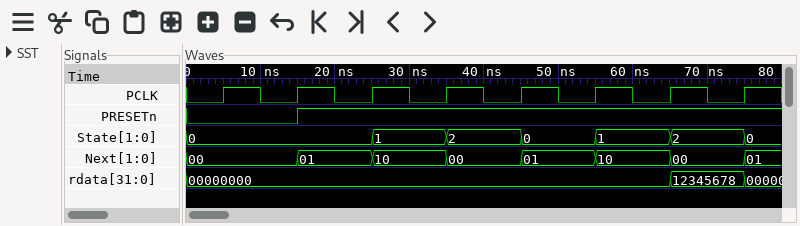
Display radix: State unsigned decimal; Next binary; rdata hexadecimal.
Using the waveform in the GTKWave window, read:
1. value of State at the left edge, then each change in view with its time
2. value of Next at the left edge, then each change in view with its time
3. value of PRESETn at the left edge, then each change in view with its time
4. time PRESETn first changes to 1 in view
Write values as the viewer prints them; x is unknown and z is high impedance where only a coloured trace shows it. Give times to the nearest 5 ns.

0, 1 at 25 ns, 2 at 35 ns, 0 at 45 ns, 1 at 55 ns, 2 at 65 ns, 0 at 75 ns
00, 01 at 15 ns, 10 at 25 ns, 00 at 35 ns, 01 at 45 ns, 10 at 55 ns, 00 at 65 ns, 01 at 75 ns
0, 1 at 15 ns
15 ns
